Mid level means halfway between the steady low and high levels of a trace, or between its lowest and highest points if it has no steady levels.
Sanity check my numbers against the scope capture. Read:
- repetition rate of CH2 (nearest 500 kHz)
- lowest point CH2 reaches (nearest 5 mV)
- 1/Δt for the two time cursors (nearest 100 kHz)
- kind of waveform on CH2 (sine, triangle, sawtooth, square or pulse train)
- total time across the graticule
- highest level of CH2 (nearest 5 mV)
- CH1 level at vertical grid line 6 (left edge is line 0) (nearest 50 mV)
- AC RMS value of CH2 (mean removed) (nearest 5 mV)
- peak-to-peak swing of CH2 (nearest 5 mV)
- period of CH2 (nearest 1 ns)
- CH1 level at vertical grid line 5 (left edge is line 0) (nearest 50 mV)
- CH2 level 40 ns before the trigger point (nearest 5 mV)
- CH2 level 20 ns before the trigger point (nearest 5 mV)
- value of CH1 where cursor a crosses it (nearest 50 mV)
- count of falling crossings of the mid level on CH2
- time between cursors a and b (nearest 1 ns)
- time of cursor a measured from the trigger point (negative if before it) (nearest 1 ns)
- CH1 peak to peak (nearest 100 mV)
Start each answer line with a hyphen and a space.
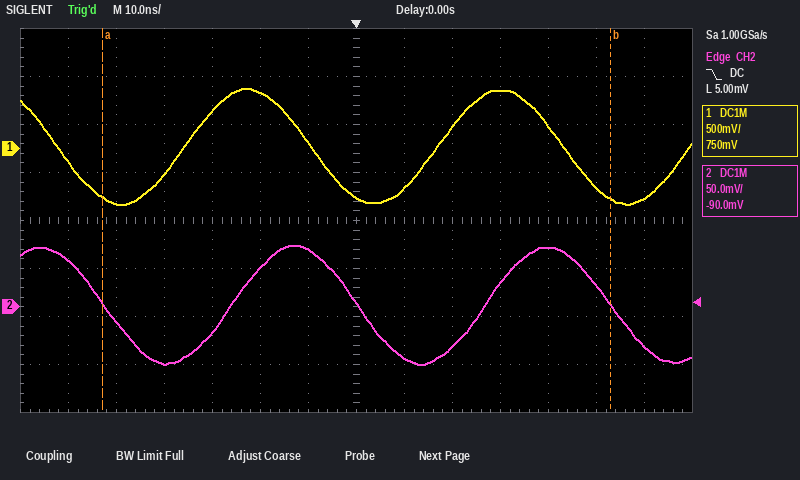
- 19.0 MHz
- -60 mV
- 9.4 MHz
- sine
- 140 ns
- 65 mV
- 50 mV
- 45 mV
- 125 mV
- 53 ns
- 600 mV
- -60 mV
- 40 mV
- -500 mV
- 3
- 106 ns
- -53 ns
- 1.20 V
